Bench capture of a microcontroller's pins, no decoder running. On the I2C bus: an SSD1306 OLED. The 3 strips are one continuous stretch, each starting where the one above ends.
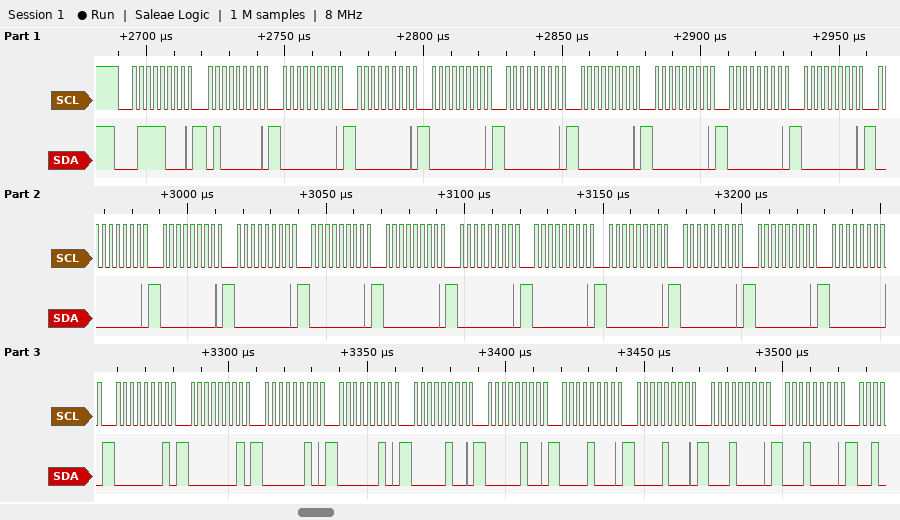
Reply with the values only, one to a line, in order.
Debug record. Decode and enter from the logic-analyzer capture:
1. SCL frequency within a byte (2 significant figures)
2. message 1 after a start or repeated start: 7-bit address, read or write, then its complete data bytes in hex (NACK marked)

400 kHz
0x3C write: 40 00 00 00 00 00 00 00 00 00 00 00 00 00 00 00 00 00 00 00 01 01 02 02 04 04 08 08 10 10
